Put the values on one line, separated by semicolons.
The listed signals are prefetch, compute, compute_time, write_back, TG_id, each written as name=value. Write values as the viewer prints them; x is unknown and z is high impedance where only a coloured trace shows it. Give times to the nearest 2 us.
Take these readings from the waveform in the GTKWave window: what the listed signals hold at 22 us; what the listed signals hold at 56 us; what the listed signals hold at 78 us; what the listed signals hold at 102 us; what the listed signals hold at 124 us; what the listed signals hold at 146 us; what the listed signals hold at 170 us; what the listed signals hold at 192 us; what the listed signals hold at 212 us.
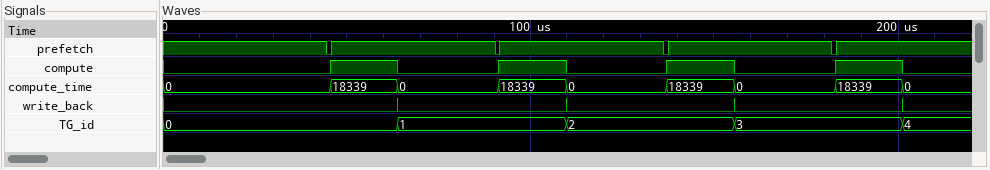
prefetch=1, compute=0, compute_time=0, write_back=0, TG_id=0; prefetch=1, compute=1, compute_time=18339, write_back=0, TG_id=0; prefetch=1, compute=0, compute_time=0, write_back=0, TG_id=1; prefetch=1, compute=1, compute_time=18339, write_back=0, TG_id=1; prefetch=1, compute=0, compute_time=0, write_back=0, TG_id=2; prefetch=1, compute=1, compute_time=18339, write_back=0, TG_id=2; prefetch=1, compute=0, compute_time=0, write_back=0, TG_id=3; prefetch=1, compute=1, compute_time=18339, write_back=0, TG_id=3; prefetch=1, compute=0, compute_time=0, write_back=0, TG_id=4
